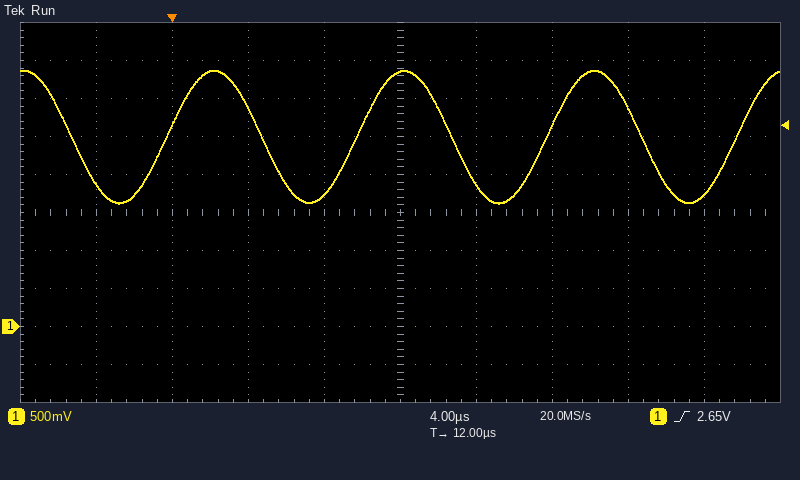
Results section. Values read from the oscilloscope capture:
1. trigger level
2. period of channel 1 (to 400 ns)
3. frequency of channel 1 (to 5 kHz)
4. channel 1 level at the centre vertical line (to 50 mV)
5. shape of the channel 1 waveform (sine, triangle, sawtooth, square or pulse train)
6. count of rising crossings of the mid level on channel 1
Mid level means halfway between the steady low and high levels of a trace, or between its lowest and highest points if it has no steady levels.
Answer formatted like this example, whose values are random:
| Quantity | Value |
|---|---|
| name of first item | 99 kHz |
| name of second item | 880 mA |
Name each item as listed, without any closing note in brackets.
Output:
| Quantity | Value |
|---|---|
| trigger level | 2.65 V |
| period of channel 1 | 10.0 µs |
| frequency of channel 1 | 100 kHz |
| channel 1 level at the centre vertical line | 3.35 V |
| shape of the channel 1 waveform | sine |
| count of rising crossings of the mid level on channel 1 | 4 |
